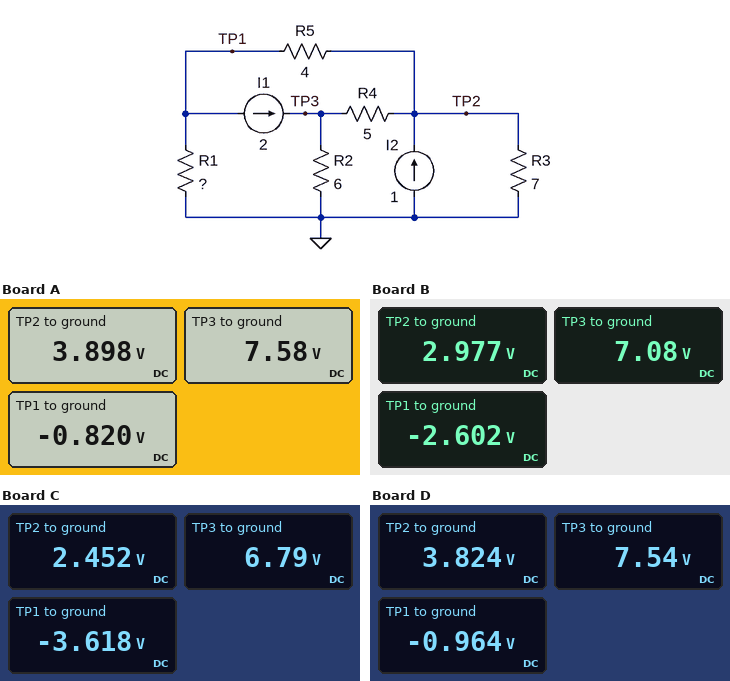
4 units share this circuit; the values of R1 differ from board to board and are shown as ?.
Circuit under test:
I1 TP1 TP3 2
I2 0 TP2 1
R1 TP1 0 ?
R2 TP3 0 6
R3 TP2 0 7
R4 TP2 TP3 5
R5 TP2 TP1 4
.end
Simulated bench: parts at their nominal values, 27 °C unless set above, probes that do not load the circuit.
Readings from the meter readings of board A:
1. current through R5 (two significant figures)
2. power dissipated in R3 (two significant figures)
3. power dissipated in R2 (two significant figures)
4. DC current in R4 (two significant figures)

1.2 A
2.2 W
9.6 W
740 mA
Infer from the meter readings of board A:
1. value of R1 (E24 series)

1 Ω
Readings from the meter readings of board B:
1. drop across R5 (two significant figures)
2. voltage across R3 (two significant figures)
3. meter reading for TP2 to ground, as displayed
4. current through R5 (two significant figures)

5.6 V
3.0 V
2.977 V
1.4 A
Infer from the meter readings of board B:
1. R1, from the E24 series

4.3 Ω
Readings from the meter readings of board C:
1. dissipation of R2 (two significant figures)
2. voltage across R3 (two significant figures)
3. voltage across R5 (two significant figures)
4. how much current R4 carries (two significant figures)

7.7 W
2.5 V
6.1 V
870 mA
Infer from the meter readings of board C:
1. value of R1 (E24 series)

7.5 Ω
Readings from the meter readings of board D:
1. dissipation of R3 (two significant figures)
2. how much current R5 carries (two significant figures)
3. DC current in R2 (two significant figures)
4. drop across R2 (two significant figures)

2.1 W
1.2 A
1.3 A
7.5 V
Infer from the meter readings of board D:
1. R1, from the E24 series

1.2 Ω
